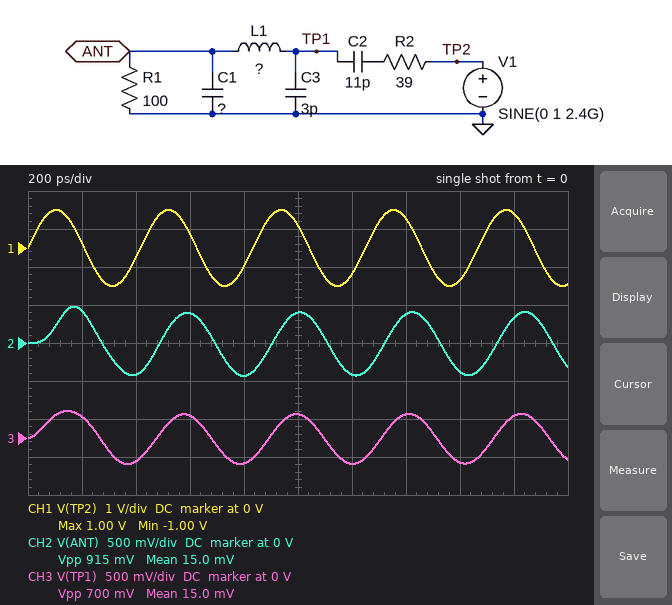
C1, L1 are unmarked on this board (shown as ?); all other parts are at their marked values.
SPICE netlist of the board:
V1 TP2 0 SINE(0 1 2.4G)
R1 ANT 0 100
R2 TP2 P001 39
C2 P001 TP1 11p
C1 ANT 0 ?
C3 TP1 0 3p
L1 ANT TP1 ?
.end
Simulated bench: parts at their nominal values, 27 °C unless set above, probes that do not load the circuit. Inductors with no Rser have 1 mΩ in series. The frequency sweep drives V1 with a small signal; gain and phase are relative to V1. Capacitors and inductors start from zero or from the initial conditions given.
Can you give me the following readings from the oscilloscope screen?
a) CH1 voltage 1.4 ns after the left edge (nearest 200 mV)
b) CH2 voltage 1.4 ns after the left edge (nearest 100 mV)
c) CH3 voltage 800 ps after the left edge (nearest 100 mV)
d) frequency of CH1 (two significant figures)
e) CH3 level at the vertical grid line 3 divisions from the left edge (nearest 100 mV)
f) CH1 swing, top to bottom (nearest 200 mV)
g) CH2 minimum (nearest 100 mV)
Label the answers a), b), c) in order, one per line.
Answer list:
a) 800 mV
b) 400 mV
c) -300 mV
d) 2.4 GHz
e) 300 mV
f) 2.0 V
g) -400 mV
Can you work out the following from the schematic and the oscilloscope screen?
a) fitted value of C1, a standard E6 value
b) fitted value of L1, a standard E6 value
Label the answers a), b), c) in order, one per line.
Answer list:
a) 1 pF
b) 1 nH
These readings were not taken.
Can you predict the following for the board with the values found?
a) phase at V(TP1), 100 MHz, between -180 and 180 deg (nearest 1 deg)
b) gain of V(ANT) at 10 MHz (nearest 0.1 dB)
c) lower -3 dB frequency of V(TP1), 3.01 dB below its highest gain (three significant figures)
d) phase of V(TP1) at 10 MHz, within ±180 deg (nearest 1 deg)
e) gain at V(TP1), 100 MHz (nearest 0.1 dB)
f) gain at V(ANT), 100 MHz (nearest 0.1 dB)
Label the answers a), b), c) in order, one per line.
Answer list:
a) 38 deg
b) -23.3 dB
c) 79.1 MHz
d) 83 deg
e) -6.9 dB
f) -6.9 dB
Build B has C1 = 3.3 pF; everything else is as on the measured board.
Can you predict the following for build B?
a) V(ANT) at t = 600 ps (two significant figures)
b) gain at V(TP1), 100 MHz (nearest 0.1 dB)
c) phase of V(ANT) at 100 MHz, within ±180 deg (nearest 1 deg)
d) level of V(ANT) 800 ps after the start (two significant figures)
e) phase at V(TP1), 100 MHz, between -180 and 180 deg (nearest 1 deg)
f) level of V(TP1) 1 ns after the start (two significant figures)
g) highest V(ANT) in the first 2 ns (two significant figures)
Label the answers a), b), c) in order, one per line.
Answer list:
a) 350 mV
b) -7.4 dB
c) 33 deg
d) -370 mV
e) 34 deg
f) 89 mV
g) 420 mV
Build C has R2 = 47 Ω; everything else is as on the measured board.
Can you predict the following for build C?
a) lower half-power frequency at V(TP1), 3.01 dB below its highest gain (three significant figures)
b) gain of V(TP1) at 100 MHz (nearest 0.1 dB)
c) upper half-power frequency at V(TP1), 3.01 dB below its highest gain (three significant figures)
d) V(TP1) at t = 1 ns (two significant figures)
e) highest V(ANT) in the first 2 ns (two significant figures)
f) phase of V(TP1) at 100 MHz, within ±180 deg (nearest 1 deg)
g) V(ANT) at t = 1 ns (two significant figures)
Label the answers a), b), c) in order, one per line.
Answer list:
a) 75.4 MHz
b) -7.1 dB
c) 1.56 GHz
d) 270 mV
e) 430 mV
f) 36 deg
g) 340 mV
